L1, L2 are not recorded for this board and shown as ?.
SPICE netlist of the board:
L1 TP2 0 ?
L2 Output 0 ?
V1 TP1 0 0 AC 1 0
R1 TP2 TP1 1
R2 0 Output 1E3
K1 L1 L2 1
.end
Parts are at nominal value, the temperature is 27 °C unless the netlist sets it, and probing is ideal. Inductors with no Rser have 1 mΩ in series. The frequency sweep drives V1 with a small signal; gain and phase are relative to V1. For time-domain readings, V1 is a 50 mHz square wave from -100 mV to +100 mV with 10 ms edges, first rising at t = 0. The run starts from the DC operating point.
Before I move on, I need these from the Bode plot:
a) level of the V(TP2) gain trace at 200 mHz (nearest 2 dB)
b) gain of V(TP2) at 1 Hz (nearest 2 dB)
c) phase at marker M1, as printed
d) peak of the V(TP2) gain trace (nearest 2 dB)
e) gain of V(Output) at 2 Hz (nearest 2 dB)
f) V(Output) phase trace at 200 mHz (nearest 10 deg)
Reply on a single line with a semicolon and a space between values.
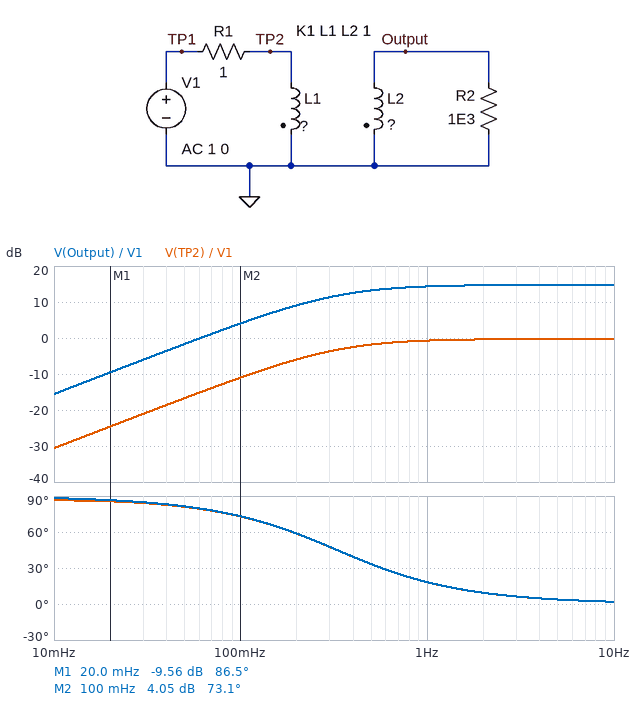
-6 dB; 0 dB; 86.5 deg; 0 dB; 14 dB; 60 deg
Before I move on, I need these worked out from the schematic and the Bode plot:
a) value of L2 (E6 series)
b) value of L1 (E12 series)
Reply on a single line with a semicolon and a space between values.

15 H; 470 mH
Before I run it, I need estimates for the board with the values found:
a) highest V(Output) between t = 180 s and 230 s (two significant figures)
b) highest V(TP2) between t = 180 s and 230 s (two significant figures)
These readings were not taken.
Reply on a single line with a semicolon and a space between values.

1.1 V; 190 mV
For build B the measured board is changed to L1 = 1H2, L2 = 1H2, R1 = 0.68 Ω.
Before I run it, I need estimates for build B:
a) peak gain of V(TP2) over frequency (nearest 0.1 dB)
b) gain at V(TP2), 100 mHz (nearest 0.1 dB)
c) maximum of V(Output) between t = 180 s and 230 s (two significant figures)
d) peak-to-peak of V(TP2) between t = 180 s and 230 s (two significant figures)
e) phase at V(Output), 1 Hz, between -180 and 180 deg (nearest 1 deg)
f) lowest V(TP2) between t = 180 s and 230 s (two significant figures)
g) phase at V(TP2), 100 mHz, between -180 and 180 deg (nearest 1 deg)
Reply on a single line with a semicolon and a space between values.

0 dB; -2.6 dB; 200 mV; 400 mV; 5 deg; -200 mV; 42 deg
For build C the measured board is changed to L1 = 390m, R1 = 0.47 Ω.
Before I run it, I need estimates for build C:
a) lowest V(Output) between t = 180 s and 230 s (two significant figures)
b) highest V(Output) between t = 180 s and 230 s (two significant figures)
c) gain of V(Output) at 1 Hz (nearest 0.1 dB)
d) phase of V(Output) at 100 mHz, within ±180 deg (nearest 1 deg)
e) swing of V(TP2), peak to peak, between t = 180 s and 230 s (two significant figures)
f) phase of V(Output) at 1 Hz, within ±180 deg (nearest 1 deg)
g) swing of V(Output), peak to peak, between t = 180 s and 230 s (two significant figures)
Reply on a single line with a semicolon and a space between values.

-1.2 V; 1.2 V; 15.5 dB; 62 deg; 390 mV; 11 deg; 2.4 V
